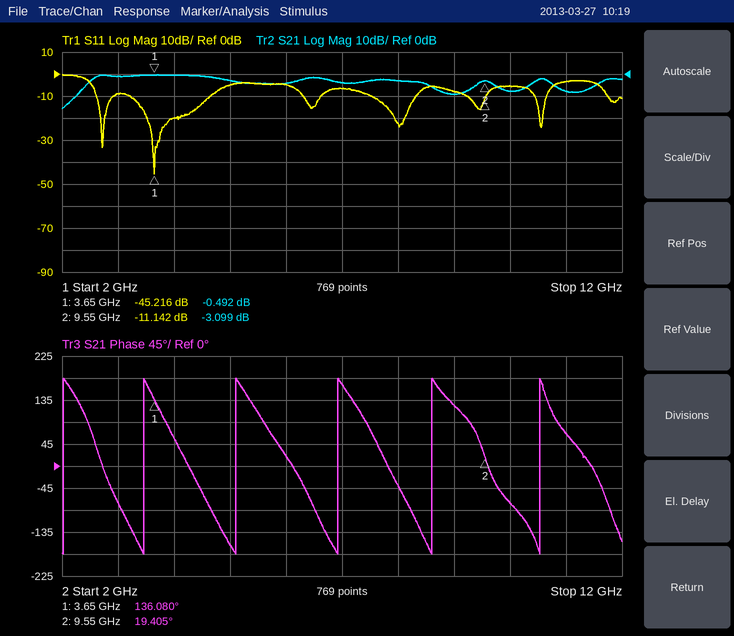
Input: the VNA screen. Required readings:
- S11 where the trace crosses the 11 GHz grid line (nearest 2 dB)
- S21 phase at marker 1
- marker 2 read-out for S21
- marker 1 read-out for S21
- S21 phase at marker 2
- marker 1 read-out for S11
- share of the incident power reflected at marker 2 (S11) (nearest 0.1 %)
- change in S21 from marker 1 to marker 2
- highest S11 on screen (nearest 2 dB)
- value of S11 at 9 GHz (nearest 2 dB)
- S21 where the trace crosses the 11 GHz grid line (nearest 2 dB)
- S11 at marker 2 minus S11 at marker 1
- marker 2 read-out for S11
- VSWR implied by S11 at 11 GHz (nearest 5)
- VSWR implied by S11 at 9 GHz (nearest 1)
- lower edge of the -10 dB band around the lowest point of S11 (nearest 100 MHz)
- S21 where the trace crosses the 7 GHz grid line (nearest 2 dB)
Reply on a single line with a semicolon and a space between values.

-4 dB; 136.080°; -3.099 dB; -0.492 dB; 19.405°; -45.216 dB; 7.7 %; -2.607 dB; 0 dB; -8 dB; -8 dB; 34.074 dB; -11.142 dB; 5; 2; 3.2 GHz; -4 dB
